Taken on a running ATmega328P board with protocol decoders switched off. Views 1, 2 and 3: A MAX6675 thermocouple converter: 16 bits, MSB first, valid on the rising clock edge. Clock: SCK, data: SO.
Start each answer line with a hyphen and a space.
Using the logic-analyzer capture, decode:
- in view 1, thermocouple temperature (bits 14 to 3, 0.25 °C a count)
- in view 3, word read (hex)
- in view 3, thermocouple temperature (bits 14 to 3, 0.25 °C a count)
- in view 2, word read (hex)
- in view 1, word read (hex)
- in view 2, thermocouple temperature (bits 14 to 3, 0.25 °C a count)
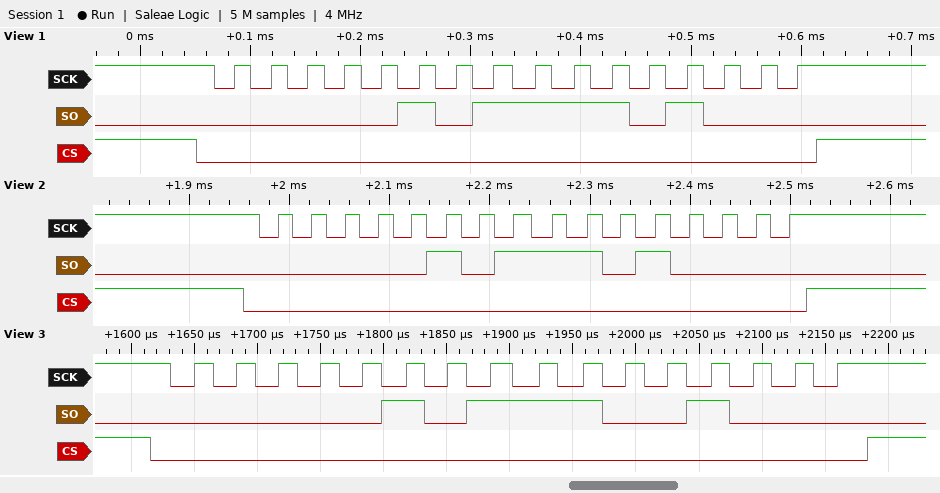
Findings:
- 47.25 °C
- 0x05C8
- 46.25 °C
- 0x05D0
- 0x05E8
- 46.50 °C
